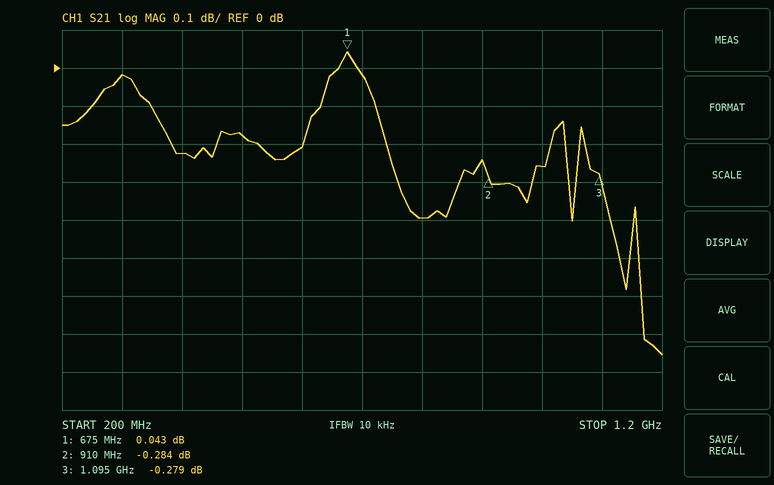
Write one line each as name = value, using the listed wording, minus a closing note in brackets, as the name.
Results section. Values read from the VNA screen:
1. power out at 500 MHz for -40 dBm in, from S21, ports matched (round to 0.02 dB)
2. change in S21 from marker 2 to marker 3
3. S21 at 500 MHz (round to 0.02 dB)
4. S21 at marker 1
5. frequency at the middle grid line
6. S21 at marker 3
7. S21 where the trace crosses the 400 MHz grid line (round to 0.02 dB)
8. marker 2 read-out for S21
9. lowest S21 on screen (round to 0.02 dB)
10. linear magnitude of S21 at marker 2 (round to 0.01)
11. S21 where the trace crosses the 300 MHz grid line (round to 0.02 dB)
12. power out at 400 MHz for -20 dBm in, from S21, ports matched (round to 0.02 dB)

power out at 500 MHz for -40 dBm in, from S21, ports matched = -40.18 dBm
change in S21 from marker 2 to marker 3 = 0.005 dB
S21 at 500 MHz = -0.18 dB
S21 at marker 1 = 0.043 dB
frequency at the middle grid line = 700 MHz
S21 at marker 3 = -0.279 dB
S21 where the trace crosses the 400 MHz grid line = -0.22 dB
marker 2 read-out for S21 = -0.284 dB
lowest S21 on screen = -0.76 dB
linear magnitude of S21 at marker 2 = 0.97
S21 where the trace crosses the 300 MHz grid line = -0.02 dB
power out at 400 MHz for -20 dBm in, from S21, ports matched = -20.22 dBm
